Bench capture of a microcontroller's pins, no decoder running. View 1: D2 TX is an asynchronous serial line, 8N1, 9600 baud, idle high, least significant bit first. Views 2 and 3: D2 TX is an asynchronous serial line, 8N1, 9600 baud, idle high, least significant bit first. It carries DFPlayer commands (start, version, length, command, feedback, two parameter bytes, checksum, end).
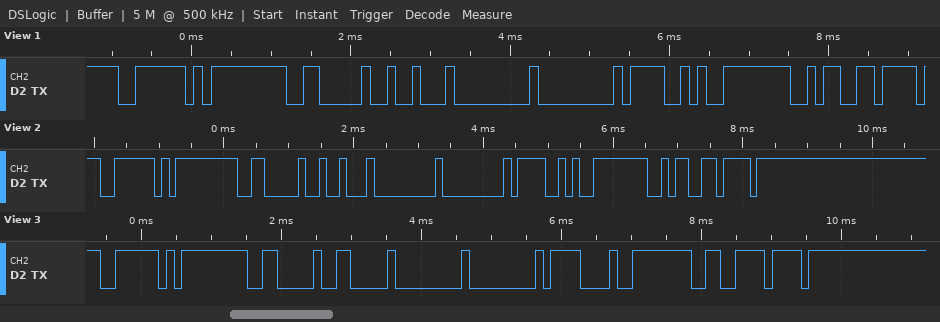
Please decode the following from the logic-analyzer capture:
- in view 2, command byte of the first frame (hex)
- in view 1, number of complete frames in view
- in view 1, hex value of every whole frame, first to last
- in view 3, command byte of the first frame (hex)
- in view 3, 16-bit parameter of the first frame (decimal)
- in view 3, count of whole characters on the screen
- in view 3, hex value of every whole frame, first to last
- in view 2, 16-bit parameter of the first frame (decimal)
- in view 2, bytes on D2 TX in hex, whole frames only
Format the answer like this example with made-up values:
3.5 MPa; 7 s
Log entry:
0x12; 9; 0x7E 0xFF 0x06 0x12 0x00 0x00 0x4F 0xFE 0x9A; 0x06; 15; 10; 7E FF 06 06 00 00 0F FE E6 EF; 79; 7E FF 06 12 00 00 4F FE 9A EF
